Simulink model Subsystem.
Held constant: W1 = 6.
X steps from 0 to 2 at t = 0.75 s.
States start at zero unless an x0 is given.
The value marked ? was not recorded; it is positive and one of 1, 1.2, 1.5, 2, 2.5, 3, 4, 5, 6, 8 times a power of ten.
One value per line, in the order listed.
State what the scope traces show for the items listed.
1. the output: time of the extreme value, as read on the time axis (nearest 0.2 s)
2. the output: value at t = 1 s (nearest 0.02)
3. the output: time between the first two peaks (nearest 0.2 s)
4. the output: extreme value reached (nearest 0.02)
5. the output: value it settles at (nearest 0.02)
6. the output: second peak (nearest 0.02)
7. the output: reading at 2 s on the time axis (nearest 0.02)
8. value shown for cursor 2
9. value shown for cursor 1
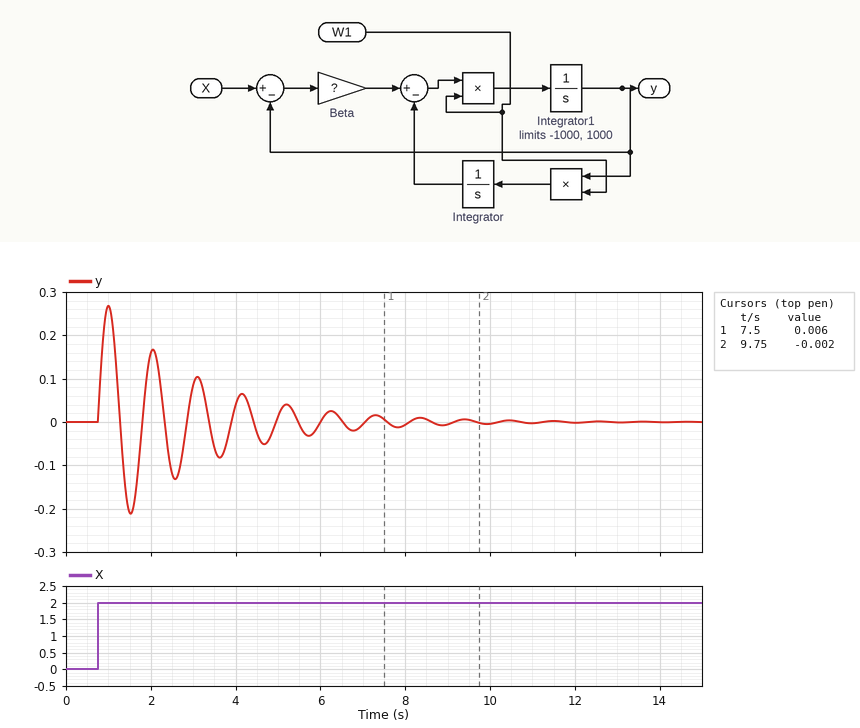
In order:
1.0 s
0.26
1.0 s
0.26
0.00
0.16
0.16
-0.002
0.006
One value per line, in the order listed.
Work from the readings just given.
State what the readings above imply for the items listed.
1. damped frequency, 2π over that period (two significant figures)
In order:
6.3 rad/s
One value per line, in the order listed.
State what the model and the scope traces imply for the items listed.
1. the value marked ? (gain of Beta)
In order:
0.15
